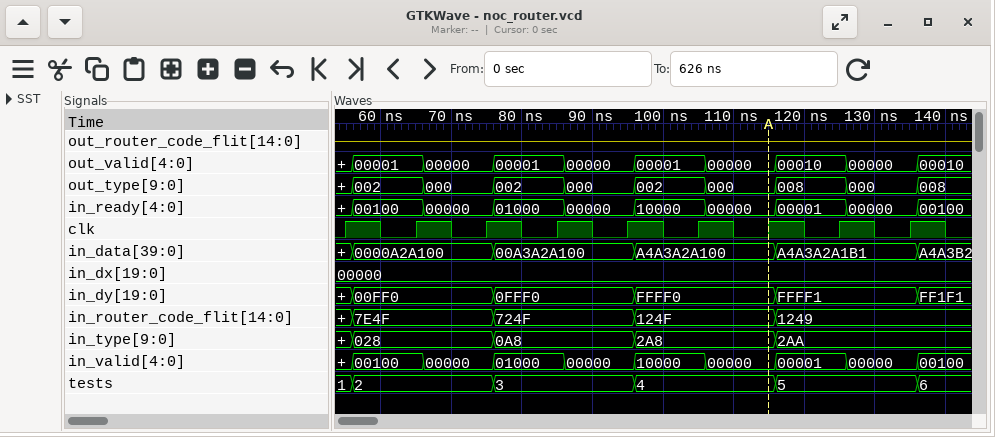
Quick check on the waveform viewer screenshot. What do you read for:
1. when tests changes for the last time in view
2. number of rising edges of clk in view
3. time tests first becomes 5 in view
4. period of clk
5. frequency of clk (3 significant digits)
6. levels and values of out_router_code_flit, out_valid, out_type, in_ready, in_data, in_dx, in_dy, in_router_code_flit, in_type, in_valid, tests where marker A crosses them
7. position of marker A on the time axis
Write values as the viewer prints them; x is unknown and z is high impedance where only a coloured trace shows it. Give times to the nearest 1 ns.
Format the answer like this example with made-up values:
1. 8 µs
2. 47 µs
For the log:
1. 136 ns
2. 9
3. 116 ns
4. 10 ns
5. 100 MHz
6. out_router_code_flit=z, out_valid=00000, out_type=000, in_ready=00000, in_data=A4A3A2A100, in_dx=00000, in_dy=FFFF0, in_router_code_flit=124F, in_type=2A8, in_valid=00000, tests=4
7. 115 ns
